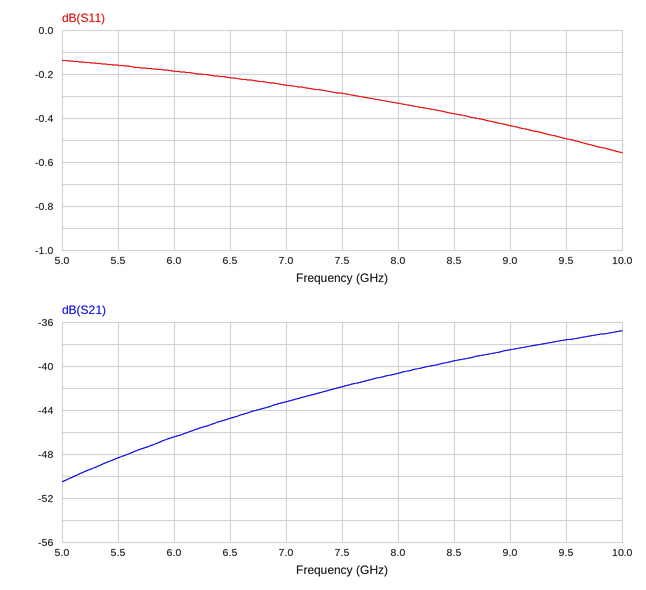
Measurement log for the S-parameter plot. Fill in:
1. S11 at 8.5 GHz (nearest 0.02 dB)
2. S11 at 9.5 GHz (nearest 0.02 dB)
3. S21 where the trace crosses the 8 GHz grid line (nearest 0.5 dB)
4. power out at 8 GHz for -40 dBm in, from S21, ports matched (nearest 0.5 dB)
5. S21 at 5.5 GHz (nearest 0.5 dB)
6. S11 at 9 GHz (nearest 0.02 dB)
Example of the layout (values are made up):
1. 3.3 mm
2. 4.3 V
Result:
1. -0.38 dB
2. -0.50 dB
3. -40.5 dB
4. -80.5 dBm
5. -48.5 dB
6. -0.44 dB
